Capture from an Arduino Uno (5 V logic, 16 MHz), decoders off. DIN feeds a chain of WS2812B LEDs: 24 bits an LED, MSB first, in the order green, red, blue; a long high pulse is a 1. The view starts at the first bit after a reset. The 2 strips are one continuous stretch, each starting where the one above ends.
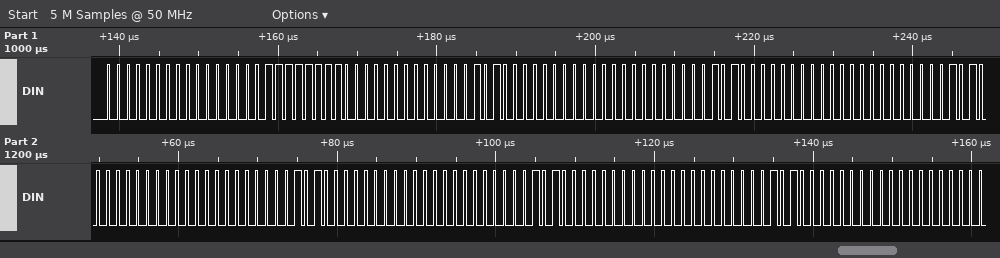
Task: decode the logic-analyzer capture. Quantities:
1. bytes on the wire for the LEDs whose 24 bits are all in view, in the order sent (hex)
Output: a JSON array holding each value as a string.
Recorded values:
["00 00 FF 00 05 00 00 05 00 00 05 00 00 05 00 00 05 00 00 05 00"]
